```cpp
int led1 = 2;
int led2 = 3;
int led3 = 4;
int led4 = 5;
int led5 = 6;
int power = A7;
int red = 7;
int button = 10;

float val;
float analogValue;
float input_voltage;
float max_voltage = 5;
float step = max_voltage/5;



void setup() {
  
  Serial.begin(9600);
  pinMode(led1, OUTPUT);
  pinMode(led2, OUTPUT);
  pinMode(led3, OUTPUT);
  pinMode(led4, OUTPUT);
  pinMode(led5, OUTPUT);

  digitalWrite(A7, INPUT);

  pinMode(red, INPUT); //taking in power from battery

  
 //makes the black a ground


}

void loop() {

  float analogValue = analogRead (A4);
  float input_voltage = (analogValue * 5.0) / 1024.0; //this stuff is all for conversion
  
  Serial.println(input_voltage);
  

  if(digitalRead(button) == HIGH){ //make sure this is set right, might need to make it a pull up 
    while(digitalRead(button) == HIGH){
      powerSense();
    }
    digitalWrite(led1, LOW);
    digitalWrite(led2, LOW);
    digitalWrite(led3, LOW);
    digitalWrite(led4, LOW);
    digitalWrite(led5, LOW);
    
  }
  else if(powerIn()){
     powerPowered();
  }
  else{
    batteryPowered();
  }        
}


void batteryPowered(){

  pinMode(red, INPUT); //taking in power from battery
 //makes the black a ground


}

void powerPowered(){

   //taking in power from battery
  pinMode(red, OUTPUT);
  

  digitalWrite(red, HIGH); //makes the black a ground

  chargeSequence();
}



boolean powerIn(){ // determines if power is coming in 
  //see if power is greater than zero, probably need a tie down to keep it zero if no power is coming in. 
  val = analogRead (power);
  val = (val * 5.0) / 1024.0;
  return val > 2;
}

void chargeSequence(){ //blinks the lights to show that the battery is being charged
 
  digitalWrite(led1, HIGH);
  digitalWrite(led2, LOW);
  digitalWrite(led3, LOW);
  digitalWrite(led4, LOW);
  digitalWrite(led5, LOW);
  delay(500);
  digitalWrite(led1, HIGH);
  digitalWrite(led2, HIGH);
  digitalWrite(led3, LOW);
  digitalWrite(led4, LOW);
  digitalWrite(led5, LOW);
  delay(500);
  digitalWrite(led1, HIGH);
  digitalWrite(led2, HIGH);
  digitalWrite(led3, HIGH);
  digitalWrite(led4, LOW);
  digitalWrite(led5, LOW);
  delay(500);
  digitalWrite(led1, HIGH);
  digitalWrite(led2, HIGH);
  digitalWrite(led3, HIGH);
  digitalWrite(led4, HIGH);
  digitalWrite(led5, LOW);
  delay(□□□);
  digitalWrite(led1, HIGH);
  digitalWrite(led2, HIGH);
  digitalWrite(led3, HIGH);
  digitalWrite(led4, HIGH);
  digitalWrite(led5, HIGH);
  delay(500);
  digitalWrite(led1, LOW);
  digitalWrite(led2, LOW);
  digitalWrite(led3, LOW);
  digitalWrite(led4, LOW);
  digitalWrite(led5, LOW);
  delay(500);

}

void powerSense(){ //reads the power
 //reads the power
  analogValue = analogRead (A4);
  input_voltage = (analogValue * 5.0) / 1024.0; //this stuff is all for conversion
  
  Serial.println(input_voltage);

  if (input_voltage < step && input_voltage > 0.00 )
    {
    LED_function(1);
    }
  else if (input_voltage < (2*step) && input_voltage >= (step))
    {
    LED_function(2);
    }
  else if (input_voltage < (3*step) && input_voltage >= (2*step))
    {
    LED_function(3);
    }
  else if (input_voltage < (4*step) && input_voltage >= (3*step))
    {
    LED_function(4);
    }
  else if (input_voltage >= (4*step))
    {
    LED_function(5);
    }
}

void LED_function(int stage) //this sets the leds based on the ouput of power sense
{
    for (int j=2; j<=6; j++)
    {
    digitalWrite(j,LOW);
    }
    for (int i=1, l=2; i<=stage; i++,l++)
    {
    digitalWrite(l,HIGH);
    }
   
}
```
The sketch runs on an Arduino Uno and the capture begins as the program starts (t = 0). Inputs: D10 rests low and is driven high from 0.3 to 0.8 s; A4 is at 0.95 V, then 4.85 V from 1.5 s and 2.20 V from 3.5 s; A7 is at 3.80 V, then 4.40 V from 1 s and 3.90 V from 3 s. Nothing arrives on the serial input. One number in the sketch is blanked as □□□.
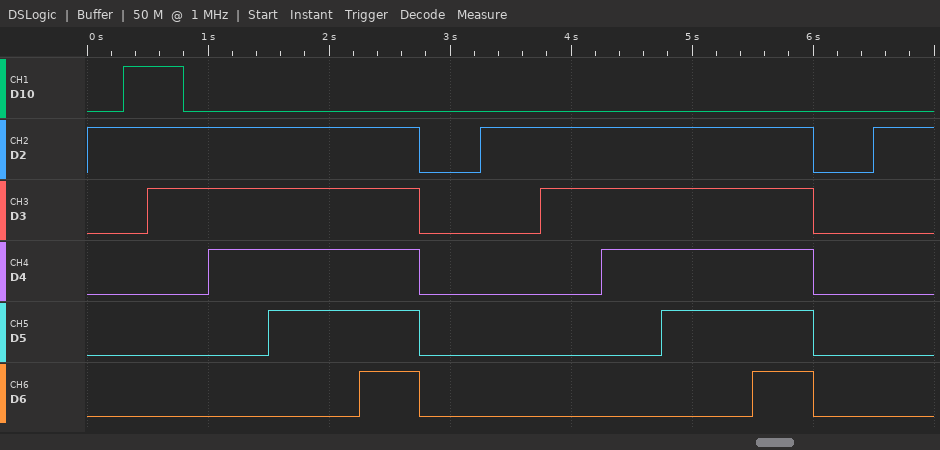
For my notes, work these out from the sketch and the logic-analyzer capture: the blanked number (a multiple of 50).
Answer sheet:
750
